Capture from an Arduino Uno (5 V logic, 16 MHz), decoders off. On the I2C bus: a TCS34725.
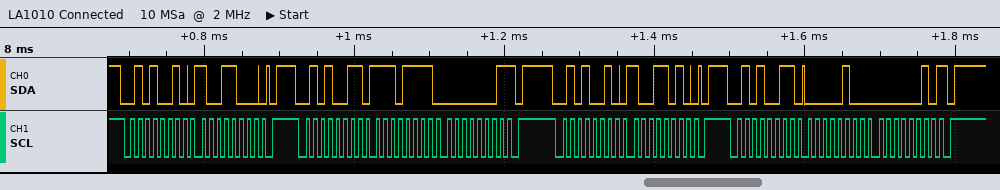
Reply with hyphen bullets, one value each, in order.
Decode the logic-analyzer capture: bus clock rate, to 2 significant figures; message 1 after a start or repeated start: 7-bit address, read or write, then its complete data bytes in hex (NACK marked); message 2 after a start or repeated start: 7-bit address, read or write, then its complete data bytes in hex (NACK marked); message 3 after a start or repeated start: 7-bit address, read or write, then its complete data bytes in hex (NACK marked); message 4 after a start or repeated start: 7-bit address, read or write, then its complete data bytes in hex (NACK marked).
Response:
- 100 kHz
- 0x29 write: 98
- 0x29 read: EF 01 NACK
- 0x29 write: 9A
- 0x29 read: 04 02 NACK
